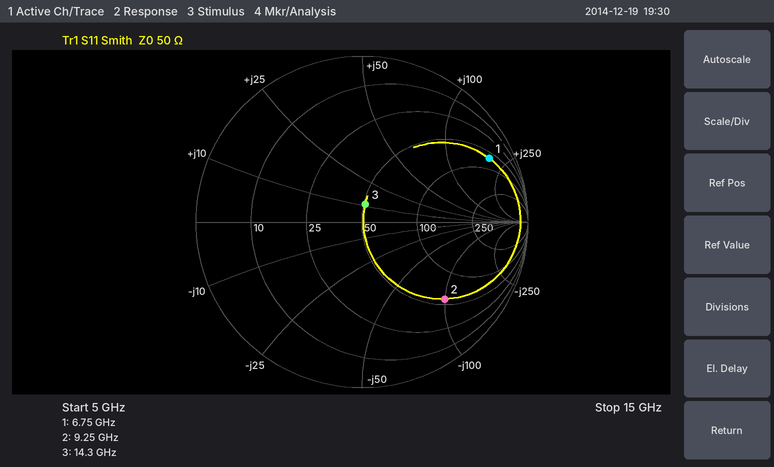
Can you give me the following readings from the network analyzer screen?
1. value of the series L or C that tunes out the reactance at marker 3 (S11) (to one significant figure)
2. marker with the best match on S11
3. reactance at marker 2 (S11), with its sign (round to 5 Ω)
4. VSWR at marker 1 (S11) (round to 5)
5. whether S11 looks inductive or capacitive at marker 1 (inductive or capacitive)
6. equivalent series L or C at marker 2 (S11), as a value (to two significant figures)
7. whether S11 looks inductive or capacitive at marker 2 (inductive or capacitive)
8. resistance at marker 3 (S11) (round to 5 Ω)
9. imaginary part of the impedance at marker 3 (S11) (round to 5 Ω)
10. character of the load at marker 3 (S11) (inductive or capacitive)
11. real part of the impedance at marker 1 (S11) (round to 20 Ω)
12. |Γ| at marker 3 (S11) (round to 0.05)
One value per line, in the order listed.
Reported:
1 pF
marker 3
-100 Ω
15
inductive
170 fF
capacitive
50 Ω
+10 Ω
inductive
60 Ω
0.10
